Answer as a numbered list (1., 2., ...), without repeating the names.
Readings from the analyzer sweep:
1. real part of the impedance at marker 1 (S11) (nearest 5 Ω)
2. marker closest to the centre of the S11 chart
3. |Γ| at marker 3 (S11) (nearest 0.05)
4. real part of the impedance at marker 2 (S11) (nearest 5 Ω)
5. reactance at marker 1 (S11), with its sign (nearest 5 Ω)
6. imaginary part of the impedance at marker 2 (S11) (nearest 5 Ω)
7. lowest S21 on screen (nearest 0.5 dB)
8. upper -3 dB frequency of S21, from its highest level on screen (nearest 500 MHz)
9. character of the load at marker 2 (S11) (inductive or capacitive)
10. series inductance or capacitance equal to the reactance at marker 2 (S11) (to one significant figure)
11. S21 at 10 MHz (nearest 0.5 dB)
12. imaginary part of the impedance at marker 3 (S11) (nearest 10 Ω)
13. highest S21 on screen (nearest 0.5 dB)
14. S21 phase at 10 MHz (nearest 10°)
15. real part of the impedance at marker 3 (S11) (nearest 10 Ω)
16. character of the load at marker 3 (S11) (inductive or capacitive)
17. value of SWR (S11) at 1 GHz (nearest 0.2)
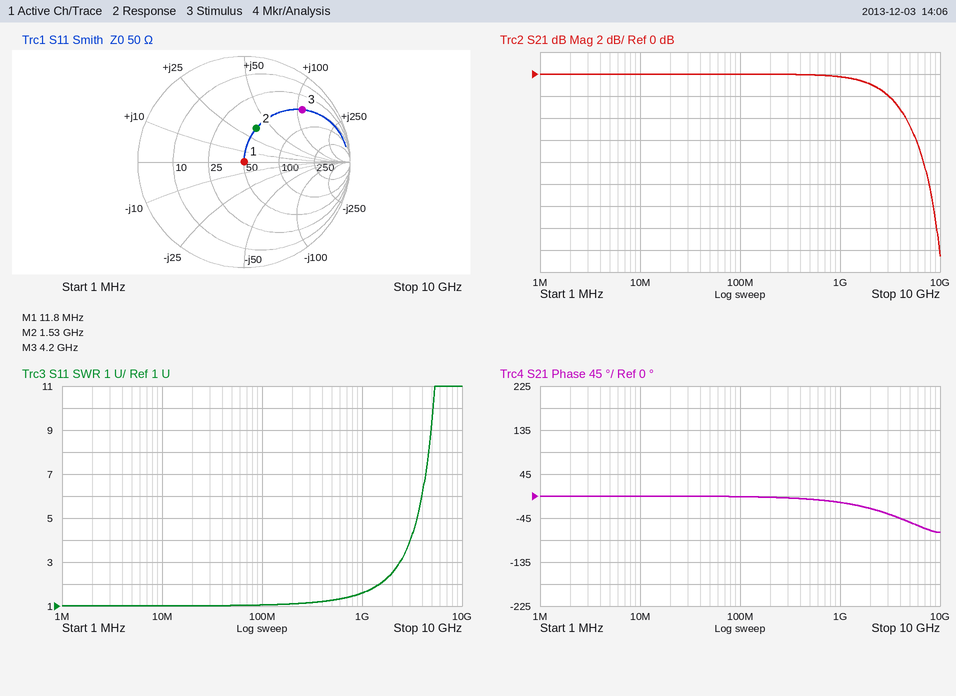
1. 50 Ω
2. marker 1
3. 0.75
4. 50 Ω
5. 0 Ω
6. +35 Ω
7. -16.5 dB
8. 4.0 GHz
9. inductive
10. 4 nH
11. 0.0 dB
12. +110 Ω
13. 0.0 dB
14. 0°
15. 50 Ω
16. inductive
17. 1.6
